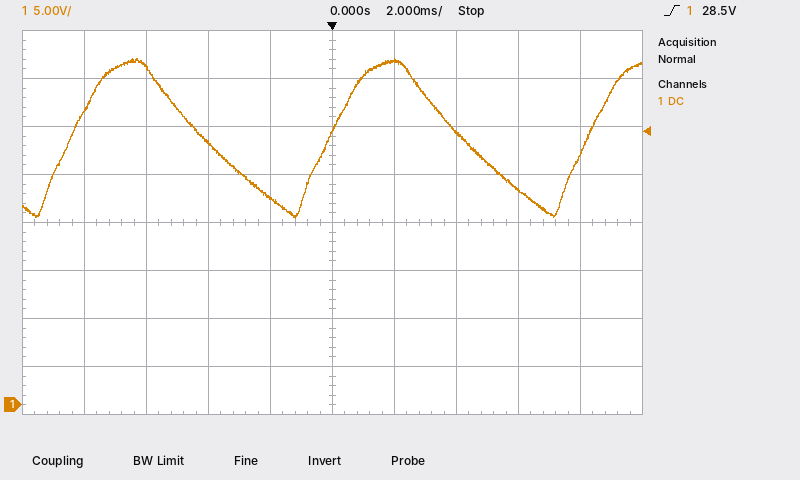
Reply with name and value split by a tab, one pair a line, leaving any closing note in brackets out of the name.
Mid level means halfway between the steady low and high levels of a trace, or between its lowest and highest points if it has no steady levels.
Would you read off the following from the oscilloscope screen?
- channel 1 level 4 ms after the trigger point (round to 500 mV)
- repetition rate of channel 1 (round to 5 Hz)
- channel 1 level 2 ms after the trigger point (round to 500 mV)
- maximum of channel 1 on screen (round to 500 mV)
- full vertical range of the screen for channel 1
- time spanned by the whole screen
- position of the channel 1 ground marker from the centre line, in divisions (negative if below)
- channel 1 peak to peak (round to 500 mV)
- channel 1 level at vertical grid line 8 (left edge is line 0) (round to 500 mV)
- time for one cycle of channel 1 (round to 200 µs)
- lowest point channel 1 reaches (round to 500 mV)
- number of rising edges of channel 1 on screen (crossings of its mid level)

channel 1 level 4 ms after the trigger point	28.5 V
repetition rate of channel 1	120 Hz
channel 1 level 2 ms after the trigger point	36.0 V
maximum of channel 1 on screen	36.0 V
full vertical range of the screen for channel 1	40 V
time spanned by the whole screen	20 ms
position of the channel 1 ground marker from the centre line, in divisions	-3.8 div
channel 1 peak to peak	16.5 V
channel 1 level at vertical grid line 8 (left edge is line 0)	22.5 V
time for one cycle of channel 1	8.4 ms
lowest point channel 1 reaches	19.5 V
number of rising edges of channel 1 on screen	3
